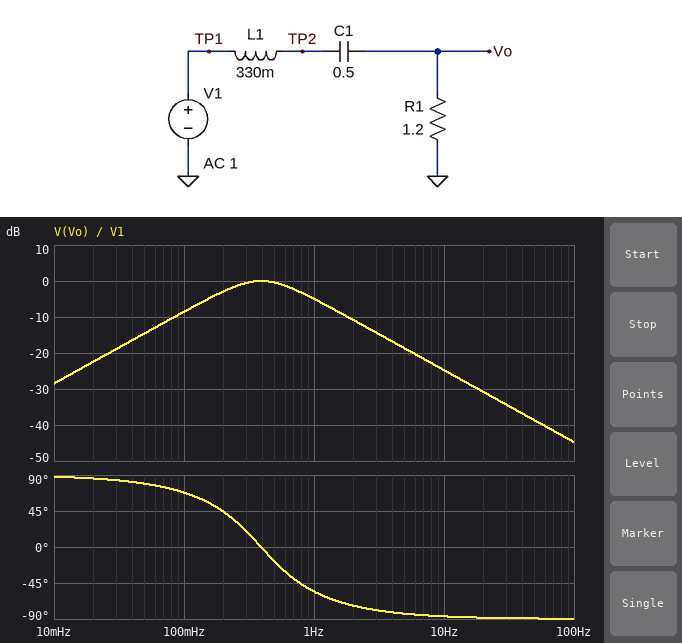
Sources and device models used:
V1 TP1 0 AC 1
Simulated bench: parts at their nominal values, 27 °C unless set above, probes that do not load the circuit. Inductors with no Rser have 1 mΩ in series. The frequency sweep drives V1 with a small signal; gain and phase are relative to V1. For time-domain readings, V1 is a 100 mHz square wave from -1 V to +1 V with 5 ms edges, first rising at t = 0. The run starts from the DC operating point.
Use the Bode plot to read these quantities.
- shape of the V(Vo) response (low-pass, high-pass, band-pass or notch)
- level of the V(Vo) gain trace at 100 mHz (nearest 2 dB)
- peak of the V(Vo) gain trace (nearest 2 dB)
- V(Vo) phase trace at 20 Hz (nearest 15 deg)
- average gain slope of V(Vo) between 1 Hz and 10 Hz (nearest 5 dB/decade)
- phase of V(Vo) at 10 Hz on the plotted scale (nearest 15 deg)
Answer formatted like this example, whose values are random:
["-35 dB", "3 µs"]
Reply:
["band-pass", "-8 dB", "0 dB", "-90 deg", "-20 dB/decade", "-90 deg"]
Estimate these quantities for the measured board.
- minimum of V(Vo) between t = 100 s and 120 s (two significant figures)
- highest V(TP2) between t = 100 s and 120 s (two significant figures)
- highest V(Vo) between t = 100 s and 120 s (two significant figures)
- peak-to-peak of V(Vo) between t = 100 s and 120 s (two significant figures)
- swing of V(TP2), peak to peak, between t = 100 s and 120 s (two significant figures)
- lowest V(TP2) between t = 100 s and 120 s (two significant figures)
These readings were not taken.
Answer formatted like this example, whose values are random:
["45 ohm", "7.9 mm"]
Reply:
["-1.3 V", "1.4 V", "1.3 V", "2.6 V", "2.8 V", "-1.4 V"]
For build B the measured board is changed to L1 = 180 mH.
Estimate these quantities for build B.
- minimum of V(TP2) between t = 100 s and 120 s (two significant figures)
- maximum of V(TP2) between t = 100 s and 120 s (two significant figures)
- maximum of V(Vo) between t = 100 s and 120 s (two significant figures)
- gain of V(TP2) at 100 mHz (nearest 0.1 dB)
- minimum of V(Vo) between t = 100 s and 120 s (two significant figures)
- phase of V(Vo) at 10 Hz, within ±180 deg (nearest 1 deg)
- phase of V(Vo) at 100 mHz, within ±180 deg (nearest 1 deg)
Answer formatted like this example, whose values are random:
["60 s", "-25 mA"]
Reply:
["-1.3 V", "1.3 V", "1.5 V", "0.3 dB", "-1.5 V", "-84 deg", "69 deg"]
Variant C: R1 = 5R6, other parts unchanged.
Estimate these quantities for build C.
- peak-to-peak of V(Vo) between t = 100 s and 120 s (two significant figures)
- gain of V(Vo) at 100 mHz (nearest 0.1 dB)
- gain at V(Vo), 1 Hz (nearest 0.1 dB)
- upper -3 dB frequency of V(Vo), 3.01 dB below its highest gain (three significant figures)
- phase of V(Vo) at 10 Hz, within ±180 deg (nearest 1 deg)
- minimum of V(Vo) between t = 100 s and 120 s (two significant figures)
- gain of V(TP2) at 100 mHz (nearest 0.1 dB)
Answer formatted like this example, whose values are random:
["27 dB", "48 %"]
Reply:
["3.2 V", "-1.1 dB", "-0.4 dB", "2.76 Hz", "-75 deg", "-1.6 V", "0.1 dB"]
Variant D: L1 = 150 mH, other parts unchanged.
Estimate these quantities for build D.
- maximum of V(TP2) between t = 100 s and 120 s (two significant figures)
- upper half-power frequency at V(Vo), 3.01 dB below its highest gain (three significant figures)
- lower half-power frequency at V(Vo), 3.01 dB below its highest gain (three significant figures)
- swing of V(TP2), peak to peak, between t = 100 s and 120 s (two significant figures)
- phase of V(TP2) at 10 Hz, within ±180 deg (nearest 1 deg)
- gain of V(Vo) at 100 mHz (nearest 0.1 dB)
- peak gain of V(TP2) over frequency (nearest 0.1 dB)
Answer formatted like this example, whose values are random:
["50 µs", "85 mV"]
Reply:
["1.2 V", "1.50 Hz", "225 mHz", "2.5 V", "-84 deg", "-8.8 dB", "1.1 dB"]
